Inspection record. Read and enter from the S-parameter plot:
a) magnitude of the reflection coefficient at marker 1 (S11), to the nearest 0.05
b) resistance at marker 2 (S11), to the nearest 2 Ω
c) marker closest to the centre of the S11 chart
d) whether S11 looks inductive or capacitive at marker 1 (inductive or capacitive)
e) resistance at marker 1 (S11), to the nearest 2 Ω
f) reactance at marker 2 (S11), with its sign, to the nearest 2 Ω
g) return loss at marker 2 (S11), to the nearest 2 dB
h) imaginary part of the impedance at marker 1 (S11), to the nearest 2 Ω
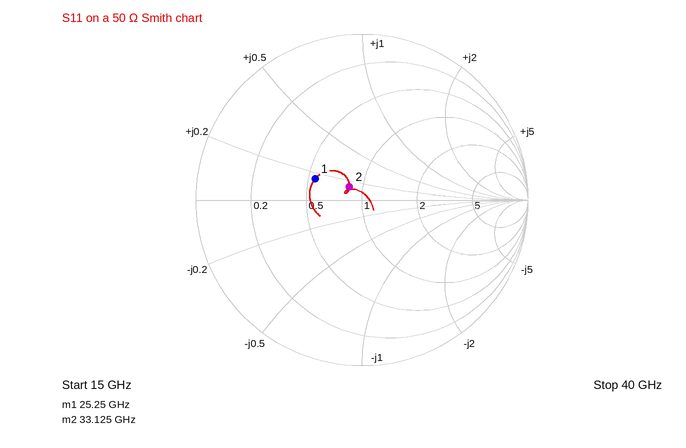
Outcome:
0.30
42 Ω
marker 2
inductive
28 Ω
+6 Ω
20 dB
+8 Ω
